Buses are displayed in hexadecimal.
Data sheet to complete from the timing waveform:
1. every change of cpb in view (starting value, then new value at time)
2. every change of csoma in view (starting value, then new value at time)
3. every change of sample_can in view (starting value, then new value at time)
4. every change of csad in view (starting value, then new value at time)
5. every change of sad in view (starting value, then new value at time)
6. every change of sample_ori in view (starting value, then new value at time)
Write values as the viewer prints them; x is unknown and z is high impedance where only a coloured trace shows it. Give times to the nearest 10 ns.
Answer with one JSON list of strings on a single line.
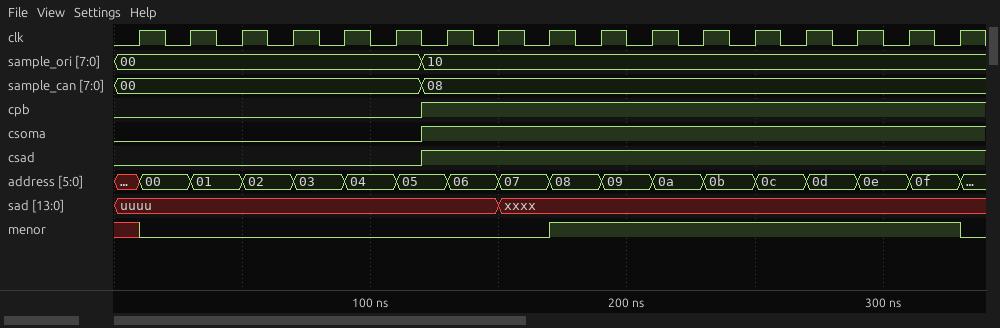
["0, 1 at 120 ns", "0, 1 at 120 ns", "00, 08 at 120 ns", "0, 1 at 120 ns", "uuuu, xxxx at 150 ns", "00, 10 at 120 ns"]
